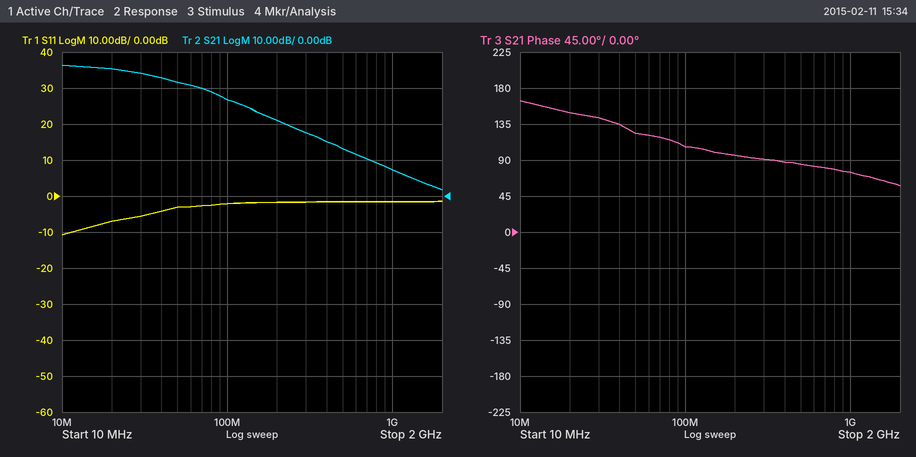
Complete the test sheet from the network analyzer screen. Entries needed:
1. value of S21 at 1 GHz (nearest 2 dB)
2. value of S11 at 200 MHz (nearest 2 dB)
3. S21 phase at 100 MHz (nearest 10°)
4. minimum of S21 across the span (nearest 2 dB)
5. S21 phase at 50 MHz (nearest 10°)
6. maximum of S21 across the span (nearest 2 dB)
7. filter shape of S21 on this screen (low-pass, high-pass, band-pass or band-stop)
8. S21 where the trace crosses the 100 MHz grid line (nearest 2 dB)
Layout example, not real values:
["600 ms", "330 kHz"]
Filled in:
["8 dB", "-2 dB", "110°", "2 dB", "120°", "36 dB", "low-pass", "26 dB"]
